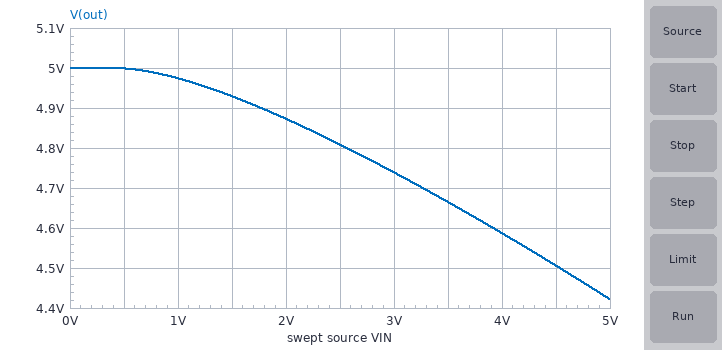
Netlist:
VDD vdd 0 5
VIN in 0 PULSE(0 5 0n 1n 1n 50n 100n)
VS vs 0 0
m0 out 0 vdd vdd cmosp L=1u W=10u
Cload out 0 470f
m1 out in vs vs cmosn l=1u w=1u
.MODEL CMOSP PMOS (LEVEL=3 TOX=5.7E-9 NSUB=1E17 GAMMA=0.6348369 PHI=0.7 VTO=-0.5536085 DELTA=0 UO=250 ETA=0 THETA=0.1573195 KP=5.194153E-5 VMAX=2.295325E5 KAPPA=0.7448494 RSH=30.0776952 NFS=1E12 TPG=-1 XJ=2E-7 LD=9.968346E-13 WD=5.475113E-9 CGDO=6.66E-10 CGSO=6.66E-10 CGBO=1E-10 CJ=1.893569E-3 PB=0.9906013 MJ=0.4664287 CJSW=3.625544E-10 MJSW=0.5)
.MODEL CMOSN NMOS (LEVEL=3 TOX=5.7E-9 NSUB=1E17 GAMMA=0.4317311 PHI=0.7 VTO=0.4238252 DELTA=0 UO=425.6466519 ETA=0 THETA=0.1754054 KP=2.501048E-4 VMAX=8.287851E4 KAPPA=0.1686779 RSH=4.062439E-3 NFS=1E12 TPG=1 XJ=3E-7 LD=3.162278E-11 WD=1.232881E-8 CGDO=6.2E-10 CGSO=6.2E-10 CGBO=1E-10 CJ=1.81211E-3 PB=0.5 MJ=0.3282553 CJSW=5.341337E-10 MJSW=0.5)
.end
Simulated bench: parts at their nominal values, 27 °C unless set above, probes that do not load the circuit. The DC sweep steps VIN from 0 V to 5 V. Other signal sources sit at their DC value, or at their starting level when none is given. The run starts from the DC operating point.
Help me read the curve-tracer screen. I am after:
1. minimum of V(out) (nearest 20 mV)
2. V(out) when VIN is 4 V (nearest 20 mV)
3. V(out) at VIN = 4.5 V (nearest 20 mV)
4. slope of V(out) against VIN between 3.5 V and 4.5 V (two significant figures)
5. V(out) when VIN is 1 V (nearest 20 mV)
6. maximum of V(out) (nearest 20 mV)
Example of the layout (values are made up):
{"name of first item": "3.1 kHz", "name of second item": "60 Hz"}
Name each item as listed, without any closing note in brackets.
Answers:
{"minimum of V(out)": "4.42 V", "V(out) when VIN is 4 V": "4.58 V", "V(out) at VIN = 4.5 V": "4.50 V", "slope of V(out) against VIN between 3.5 V and 4.5 V": "-0.16 V/V", "V(out) when VIN is 1 V": "4.98 V", "maximum of V(out)": "5.00 V"}
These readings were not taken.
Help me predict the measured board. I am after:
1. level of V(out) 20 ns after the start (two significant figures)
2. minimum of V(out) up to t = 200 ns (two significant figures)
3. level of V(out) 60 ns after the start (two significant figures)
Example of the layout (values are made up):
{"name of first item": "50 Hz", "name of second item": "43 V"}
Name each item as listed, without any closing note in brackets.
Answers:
{"level of V(out) 20 ns after the start": "4.4 V", "minimum of V(out) up to t = 200 ns": "4.4 V", "level of V(out) 60 ns after the start": "5.0 V"}
